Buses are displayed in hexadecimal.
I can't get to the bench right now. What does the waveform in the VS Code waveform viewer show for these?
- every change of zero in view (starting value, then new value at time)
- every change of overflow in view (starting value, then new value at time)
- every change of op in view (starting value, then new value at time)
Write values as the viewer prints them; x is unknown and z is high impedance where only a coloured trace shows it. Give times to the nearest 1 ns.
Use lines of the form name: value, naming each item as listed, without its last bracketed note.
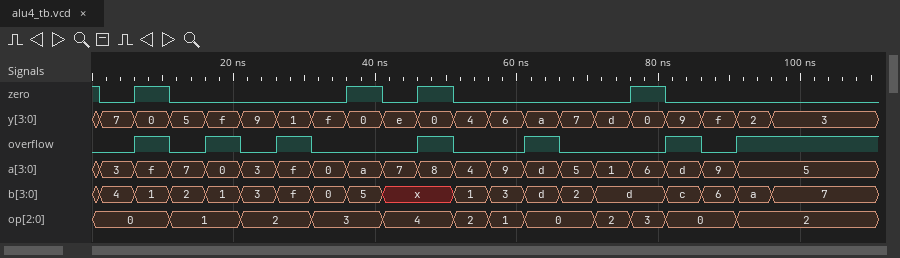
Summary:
every change of zero in view: 1, 0 at 1 ns, 1 at 6 ns, 0 at 11 ns, 1 at 36 ns, 0 at 41 ns, 1 at 46 ns, 0 at 51 ns, 1 at 76 ns, 0 at 81 ns
every change of overflow in view: 0, 1 at 6 ns, 0 at 11 ns, 1 at 16 ns, 0 at 21 ns, 1 at 26 ns, 0 at 31 ns, 1 at 46 ns, 0 at 51 ns, 1 at 61 ns, 0 at 66 ns, 1 at 81 ns, 0 at 86 ns, 1 at 91 ns
every change of op in view: 0, 1 at 11 ns, 2 at 21 ns, 3 at 31 ns, 4 at 41 ns, 2 at 51 ns, 1 at 56 ns, 0 at 61 ns, 2 at 71 ns, 3 at 76 ns, 0 at 81 ns, 2 at 91 ns
